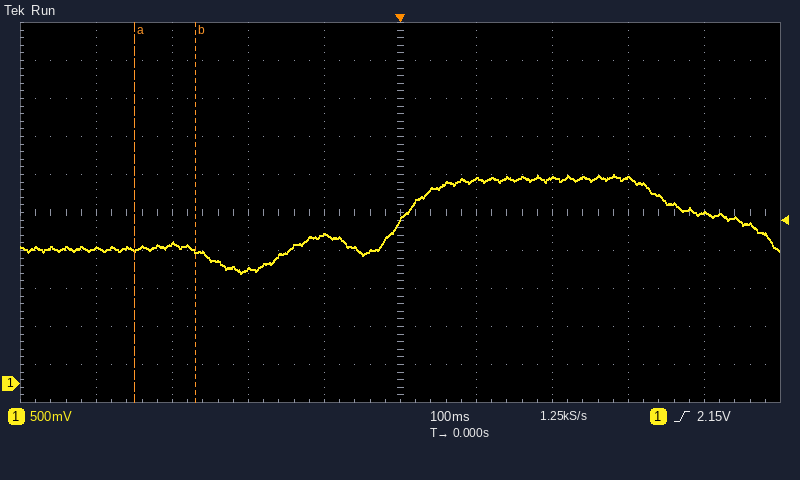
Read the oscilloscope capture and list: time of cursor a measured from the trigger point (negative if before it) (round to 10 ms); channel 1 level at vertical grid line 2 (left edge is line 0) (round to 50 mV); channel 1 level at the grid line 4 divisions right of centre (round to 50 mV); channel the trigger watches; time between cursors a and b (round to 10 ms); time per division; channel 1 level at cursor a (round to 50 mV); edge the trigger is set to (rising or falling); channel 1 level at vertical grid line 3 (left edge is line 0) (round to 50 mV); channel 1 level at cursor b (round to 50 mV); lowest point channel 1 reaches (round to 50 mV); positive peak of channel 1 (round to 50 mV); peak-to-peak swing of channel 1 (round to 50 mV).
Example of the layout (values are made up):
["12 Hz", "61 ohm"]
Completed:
["-350 ms", "1.85 V", "2.25 V", "channel 1", "80 ms", "100 ms", "1.75 V", "rising", "1.50 V", "1.75 V", "1.45 V", "2.75 V", "1.30 V"]
